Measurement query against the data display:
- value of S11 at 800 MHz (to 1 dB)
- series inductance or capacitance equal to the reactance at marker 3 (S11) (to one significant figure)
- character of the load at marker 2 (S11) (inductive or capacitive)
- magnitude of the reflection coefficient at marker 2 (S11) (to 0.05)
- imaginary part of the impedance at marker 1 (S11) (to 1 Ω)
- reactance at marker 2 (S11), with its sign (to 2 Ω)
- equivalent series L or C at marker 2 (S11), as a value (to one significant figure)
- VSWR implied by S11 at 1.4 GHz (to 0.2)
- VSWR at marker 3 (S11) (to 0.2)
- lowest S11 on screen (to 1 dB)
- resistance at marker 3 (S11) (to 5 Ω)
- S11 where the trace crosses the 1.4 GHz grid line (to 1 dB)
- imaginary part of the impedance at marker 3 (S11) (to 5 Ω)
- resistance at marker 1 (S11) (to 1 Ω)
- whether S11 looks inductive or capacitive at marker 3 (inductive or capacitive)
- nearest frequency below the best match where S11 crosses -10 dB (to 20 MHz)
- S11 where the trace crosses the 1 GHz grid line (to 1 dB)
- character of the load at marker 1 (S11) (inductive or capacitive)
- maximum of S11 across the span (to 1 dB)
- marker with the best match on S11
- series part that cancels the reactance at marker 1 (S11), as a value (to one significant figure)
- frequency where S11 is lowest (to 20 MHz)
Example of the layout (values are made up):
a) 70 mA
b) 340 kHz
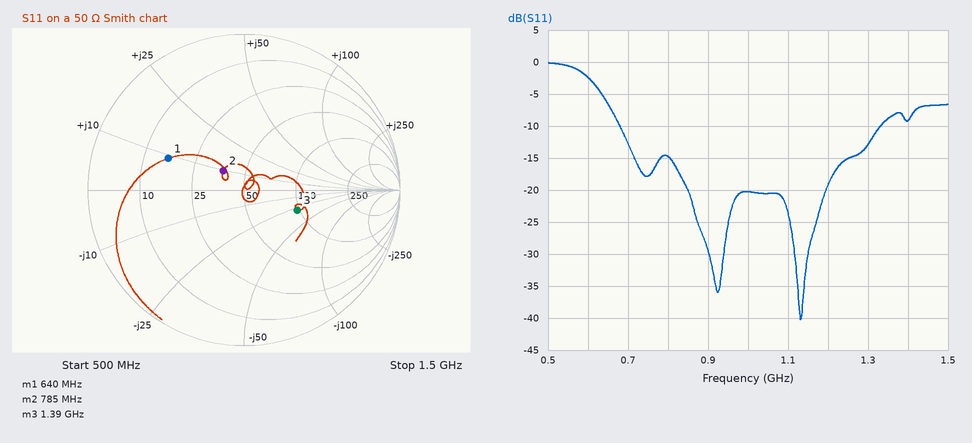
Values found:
a) -15 dB
b) 4 pF
c) inductive
d) 0.20
e) +9 Ω
f) +10 Ω
g) 2 nH
h) 2.0
i) 2.2
j) -40 dB
k) 95 Ω
l) -9 dB
m) -30 Ω
n) 16 Ω
o) capacitive
p) 680 MHz
q) -20 dB
r) inductive
s) 0 dB
t) marker 2
u) 30 pF
v) 1.14 GHz
